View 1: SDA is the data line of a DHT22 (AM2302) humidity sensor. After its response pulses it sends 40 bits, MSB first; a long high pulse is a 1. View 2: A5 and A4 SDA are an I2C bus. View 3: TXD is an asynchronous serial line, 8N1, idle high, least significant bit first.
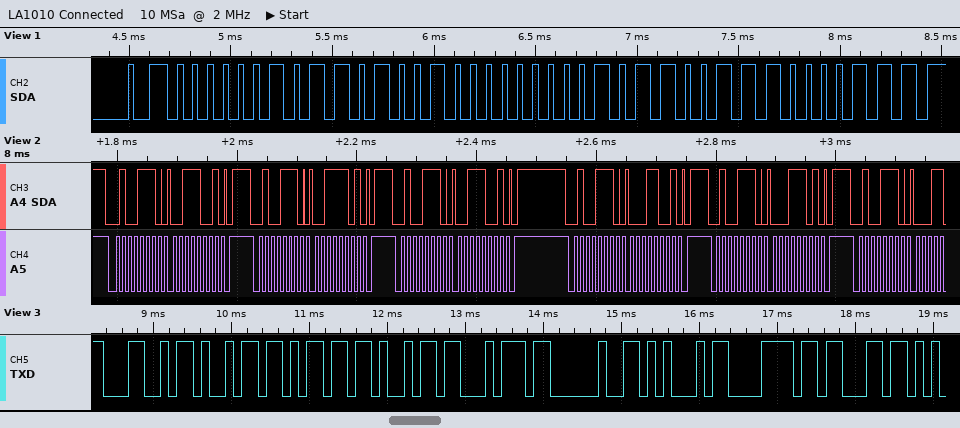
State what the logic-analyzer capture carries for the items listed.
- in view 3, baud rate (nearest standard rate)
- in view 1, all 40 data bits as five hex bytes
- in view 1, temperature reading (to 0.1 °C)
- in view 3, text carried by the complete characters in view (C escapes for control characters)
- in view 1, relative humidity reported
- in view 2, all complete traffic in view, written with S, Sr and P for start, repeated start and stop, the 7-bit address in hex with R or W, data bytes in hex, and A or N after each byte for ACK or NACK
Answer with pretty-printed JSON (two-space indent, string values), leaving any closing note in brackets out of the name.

{
  "in view 3, baud rate": "9600 baud",
  "in view 1, all 40 data bits as five hex bytes": "02 D2 00 B3 87",
  "in view 1, temperature reading": "17.9 °C",
  "in view 3, text carried by the complete characters in view": "\"Limit Exc\"",
  "in view 1, relative humidity reported": "72.2 %",
  "in view 2, all complete traffic in view, written with S, Sr and P for start, repeated start and stop, the 7-bit address in hex with R or W, data bytes in hex, and A or N after each byte for ACK or NACK": "S 27W A 39 A P S 27W A 3D A P S 27W A 39 A P S 27W A 19 A P S 27W A 1D A P S 27W A"
}
